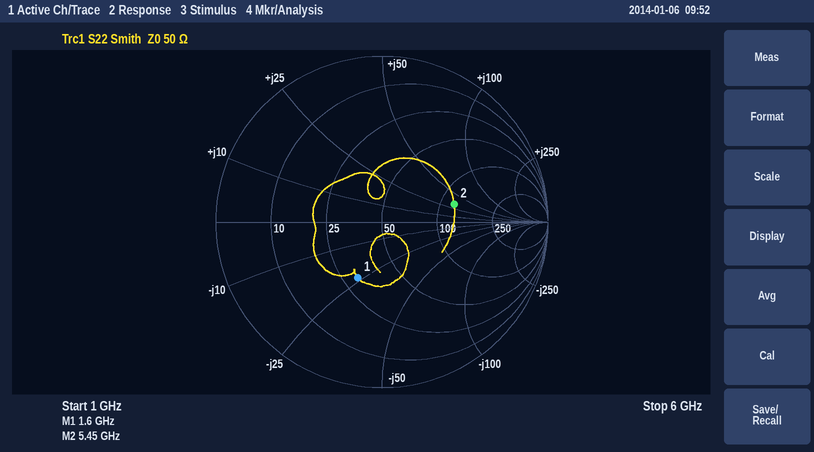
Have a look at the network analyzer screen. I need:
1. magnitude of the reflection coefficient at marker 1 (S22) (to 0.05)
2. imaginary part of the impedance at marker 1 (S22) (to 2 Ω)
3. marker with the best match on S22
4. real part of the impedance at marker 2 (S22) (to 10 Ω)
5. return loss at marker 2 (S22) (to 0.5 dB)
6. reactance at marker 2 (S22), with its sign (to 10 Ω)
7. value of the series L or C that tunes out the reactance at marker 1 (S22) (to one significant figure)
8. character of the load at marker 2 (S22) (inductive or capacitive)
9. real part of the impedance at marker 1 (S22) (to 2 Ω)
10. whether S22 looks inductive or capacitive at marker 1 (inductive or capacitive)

0.35
-24 Ω
marker 1
120 Ω
7.0 dB
+30 Ω
2 nH
inductive
30 Ω
capacitive
